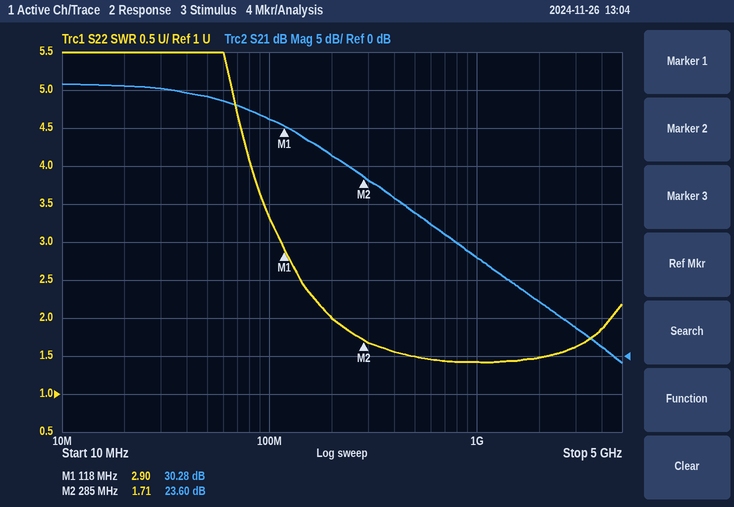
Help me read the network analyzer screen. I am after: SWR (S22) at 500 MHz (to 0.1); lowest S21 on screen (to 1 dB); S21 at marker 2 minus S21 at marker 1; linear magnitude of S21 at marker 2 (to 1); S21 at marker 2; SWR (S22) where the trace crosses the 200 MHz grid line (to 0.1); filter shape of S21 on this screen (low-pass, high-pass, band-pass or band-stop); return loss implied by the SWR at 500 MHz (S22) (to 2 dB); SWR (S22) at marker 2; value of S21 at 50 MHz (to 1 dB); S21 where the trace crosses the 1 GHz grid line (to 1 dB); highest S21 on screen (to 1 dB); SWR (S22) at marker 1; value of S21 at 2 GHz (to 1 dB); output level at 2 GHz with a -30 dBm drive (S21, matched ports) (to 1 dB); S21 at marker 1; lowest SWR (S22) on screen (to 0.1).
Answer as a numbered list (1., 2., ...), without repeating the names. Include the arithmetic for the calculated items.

1. 1.5
2. -1 dB
3. 23.6 − (30.28) = -6.68 dB
4. 10^(23.6/20) ≈ 15
5. 23.60 dB
6. 2.0
7. low-pass
8. −20 log10((1.5 − 1)/(1.5 + 1)) ≈ 14 dB
9. 1.71
10. 34 dB
11. 13 dB
12. 36 dB
13. 2.90
14. 7 dB
15. -30 dBm + (7 dB) = -23 dBm
16. 30.28 dB
17. 1.4
